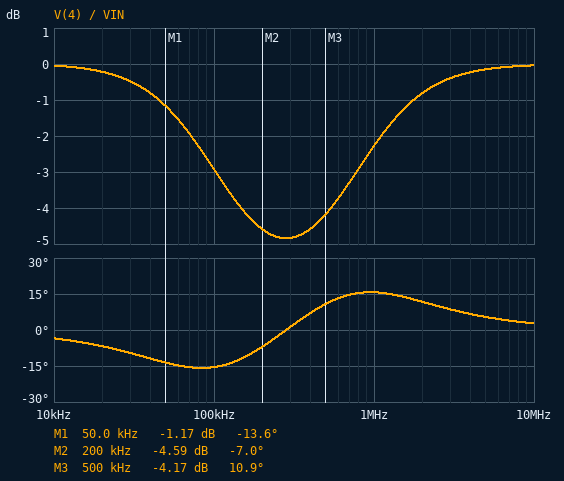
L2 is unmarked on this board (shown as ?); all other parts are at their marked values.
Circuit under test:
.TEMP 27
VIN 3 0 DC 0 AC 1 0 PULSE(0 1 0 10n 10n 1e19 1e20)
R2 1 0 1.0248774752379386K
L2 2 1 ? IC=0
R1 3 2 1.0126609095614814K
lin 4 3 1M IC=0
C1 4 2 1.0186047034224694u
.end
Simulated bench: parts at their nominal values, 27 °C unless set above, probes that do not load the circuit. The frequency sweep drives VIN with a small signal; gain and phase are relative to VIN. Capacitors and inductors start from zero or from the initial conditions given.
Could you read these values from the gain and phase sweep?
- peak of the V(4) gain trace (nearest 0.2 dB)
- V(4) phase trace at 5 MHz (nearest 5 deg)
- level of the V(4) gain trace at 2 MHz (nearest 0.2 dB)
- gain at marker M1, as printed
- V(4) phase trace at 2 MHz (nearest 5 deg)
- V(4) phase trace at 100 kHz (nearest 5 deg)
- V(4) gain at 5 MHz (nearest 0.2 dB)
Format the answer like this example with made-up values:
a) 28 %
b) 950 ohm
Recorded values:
a) 0 dB
b) 5 deg
c) -0.8 dB
d) -1.17 dB
e) 10 deg
f) -15 deg
g) -0.2 dB
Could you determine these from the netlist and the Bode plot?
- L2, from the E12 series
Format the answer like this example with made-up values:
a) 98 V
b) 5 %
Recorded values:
a) 330 µH
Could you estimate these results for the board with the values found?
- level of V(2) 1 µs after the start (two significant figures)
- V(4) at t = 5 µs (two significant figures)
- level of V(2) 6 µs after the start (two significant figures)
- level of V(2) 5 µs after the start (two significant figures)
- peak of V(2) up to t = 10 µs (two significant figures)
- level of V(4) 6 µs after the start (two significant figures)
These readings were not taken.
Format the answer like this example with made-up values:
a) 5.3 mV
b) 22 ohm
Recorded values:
a) 690 mV
b) 950 mV
c) 970 mV
d) 950 mV
e) 990 mV
f) 970 mV
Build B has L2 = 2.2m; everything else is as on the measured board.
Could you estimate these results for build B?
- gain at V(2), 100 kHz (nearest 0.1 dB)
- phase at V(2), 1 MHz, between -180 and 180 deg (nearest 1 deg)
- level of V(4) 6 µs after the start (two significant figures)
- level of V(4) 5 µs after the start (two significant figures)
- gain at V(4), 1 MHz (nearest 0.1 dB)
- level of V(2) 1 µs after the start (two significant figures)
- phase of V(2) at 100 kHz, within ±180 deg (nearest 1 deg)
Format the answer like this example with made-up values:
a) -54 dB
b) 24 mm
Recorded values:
a) -2.3 dB
b) 4 deg
c) 940 mV
d) 920 mV
e) -0.2 dB
f) 810 mV
g) -1 deg
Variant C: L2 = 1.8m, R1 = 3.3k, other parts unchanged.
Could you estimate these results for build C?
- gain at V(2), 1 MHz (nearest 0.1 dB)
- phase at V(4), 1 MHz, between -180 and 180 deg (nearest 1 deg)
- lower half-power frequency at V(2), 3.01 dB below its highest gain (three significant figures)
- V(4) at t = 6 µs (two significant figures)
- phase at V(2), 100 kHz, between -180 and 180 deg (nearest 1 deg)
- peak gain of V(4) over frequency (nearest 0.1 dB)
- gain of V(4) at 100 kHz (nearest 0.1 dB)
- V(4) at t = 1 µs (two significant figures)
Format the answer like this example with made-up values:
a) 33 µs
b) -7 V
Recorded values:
a) -1.3 dB
b) 11 deg
c) 188 Hz
d) 960 mV
e) -9 deg
f) 0 dB
g) -2.7 dB
h) 740 mV
